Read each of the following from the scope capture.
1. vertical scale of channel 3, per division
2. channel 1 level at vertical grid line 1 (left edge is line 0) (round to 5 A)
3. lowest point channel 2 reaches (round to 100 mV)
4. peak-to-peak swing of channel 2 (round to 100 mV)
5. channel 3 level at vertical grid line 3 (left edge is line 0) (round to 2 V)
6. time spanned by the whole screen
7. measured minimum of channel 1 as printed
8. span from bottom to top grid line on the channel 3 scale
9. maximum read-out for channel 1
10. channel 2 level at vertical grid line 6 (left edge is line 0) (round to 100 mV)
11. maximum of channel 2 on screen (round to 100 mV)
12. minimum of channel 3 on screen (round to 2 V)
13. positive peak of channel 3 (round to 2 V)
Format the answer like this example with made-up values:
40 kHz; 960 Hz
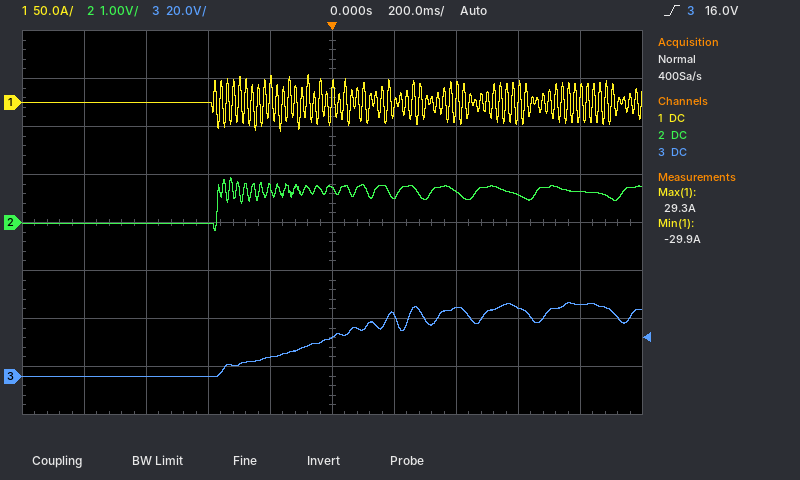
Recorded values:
20 V; 0 A; -200 mV; 1.1 V; 0 V; 2 s; -29.9 A; 160 V; 29.3 A; 500 mV; 900 mV; 0 V; 30 V
